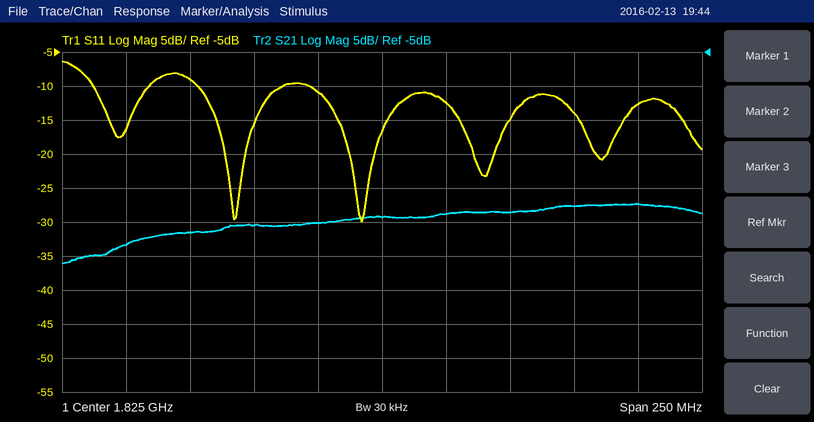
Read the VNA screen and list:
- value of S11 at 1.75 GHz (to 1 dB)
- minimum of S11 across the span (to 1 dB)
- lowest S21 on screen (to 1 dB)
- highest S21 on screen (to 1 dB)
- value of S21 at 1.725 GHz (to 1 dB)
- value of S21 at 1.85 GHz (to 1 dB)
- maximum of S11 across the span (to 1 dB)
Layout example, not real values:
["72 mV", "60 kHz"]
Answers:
["-9 dB", "-30 dB", "-36 dB", "-27 dB", "-33 dB", "-29 dB", "-6 dB"]
